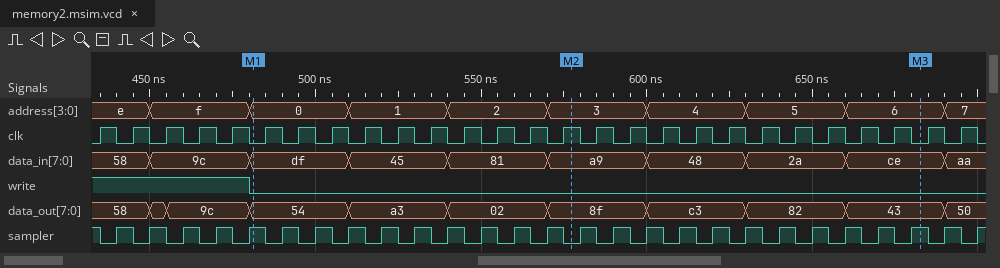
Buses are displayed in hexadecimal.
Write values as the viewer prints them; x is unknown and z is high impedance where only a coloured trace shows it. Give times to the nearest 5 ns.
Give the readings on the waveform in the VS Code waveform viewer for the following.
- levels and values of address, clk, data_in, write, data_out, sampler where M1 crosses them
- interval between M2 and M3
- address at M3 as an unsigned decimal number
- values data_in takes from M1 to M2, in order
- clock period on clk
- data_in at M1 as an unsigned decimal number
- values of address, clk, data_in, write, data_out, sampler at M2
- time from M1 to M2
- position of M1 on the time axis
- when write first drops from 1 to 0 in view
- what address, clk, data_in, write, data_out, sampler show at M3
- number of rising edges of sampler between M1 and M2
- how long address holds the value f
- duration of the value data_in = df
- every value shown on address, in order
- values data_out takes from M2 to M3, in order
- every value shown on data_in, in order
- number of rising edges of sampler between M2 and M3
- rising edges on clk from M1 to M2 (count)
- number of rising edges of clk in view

address=0, clk=0, data_in=df, write=0, data_out=54, sampler=1
105 ns
6
df, 45, 81, a9
10 ns
223
address=3, clk=1, data_in=a9, write=0, data_out=8f, sampler=0
95 ns
480 ns
480 ns
address=6, clk=0, data_in=ce, write=0, data_out=43, sampler=1
9
30 ns
30 ns
e, f, 0, 1, 2, 3, 4, 5, 6, 7
8f, c3, 82, 43
58, 9c, df, 45, 81, a9, 48, 2a, ce, aa
11
10
27
